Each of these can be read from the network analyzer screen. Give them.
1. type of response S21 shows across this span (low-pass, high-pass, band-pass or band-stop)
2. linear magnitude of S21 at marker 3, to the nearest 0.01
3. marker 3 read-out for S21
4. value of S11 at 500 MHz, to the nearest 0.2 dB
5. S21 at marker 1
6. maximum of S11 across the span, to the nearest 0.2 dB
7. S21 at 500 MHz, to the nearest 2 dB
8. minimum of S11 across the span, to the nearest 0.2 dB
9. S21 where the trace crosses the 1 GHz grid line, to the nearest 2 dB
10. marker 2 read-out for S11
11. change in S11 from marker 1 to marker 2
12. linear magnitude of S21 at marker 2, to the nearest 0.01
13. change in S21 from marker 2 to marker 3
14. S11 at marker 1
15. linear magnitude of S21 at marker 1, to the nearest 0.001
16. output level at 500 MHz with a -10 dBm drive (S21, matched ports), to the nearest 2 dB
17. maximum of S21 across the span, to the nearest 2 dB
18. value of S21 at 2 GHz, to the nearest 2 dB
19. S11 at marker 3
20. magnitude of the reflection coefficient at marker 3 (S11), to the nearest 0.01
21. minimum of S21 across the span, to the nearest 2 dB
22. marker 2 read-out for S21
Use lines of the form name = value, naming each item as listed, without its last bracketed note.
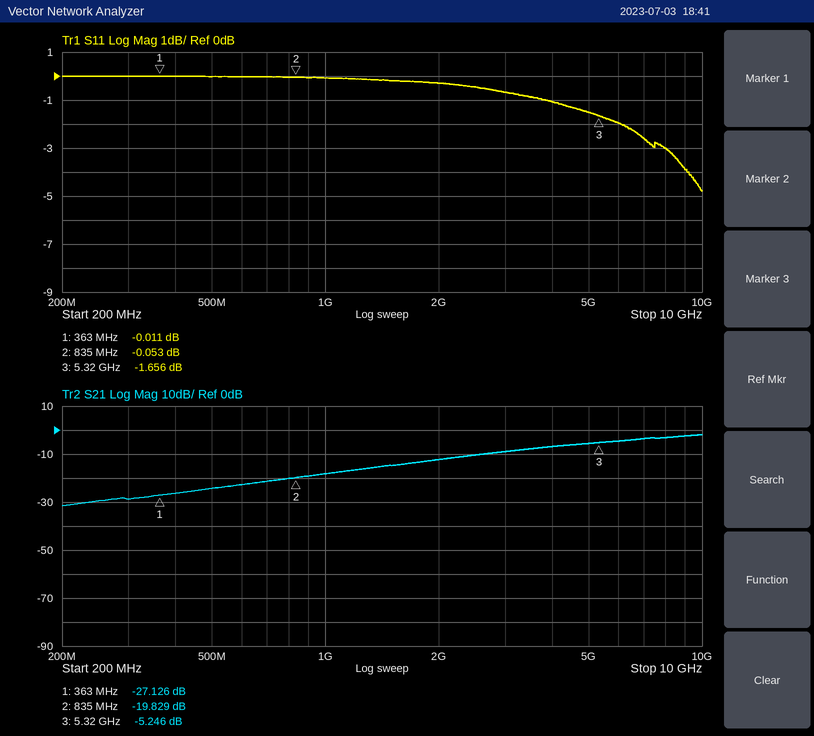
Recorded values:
type of response S21 shows across this span = high-pass
linear magnitude of S21 at marker 3, to the nearest 0.01 = 0.55
marker 3 read-out for S21 = -5.246 dB
value of S11 at 500 MHz, to the nearest 0.2 dB = 0.0 dB
S21 at marker 1 = -27.126 dB
maximum of S11 across the span, to the nearest 0.2 dB = 0.0 dB
S21 at 500 MHz, to the nearest 2 dB = -24 dB
minimum of S11 across the span, to the nearest 0.2 dB = -4.8 dB
S21 where the trace crosses the 1 GHz grid line, to the nearest 2 dB = -18 dB
marker 2 read-out for S11 = -0.053 dB
change in S11 from marker 1 to marker 2 = -0.042 dB
linear magnitude of S21 at marker 2, to the nearest 0.01 = 0.10
change in S21 from marker 2 to marker 3 = 14.583 dB
S11 at marker 1 = -0.011 dB
linear magnitude of S21 at marker 1, to the nearest 0.001 = 0.044
output level at 500 MHz with a -10 dBm drive (S21, matched ports), to the nearest 2 dB = -34 dBm
maximum of S21 across the span, to the nearest 2 dB = -2 dB
value of S21 at 2 GHz, to the nearest 2 dB = -12 dB
S11 at marker 3 = -1.656 dB
magnitude of the reflection coefficient at marker 3 (S11), to the nearest 0.01 = 0.83
minimum of S21 across the span, to the nearest 2 dB = -32 dB
marker 2 read-out for S21 = -19.829 dB
